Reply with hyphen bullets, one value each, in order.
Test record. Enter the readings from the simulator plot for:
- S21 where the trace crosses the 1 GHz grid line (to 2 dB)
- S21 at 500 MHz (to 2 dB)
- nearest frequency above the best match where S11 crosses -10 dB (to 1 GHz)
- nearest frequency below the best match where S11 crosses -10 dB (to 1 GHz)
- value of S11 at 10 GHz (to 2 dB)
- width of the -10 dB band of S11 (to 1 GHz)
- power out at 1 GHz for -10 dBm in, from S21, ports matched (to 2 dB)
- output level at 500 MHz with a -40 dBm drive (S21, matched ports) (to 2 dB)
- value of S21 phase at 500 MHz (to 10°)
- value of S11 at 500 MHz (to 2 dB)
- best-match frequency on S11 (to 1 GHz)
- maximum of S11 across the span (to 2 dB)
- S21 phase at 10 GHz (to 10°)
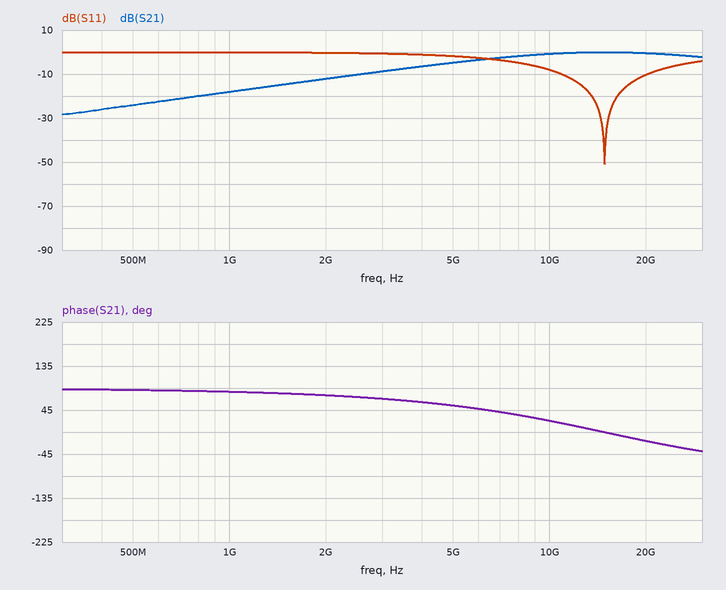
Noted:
- -18 dB
- -24 dB
- 20 GHz
- 11 GHz
- -8 dB
- 9 GHz
- -28 dBm
- -64 dBm
- 90°
- 0 dB
- 15 GHz
- 0 dB
- 20°
